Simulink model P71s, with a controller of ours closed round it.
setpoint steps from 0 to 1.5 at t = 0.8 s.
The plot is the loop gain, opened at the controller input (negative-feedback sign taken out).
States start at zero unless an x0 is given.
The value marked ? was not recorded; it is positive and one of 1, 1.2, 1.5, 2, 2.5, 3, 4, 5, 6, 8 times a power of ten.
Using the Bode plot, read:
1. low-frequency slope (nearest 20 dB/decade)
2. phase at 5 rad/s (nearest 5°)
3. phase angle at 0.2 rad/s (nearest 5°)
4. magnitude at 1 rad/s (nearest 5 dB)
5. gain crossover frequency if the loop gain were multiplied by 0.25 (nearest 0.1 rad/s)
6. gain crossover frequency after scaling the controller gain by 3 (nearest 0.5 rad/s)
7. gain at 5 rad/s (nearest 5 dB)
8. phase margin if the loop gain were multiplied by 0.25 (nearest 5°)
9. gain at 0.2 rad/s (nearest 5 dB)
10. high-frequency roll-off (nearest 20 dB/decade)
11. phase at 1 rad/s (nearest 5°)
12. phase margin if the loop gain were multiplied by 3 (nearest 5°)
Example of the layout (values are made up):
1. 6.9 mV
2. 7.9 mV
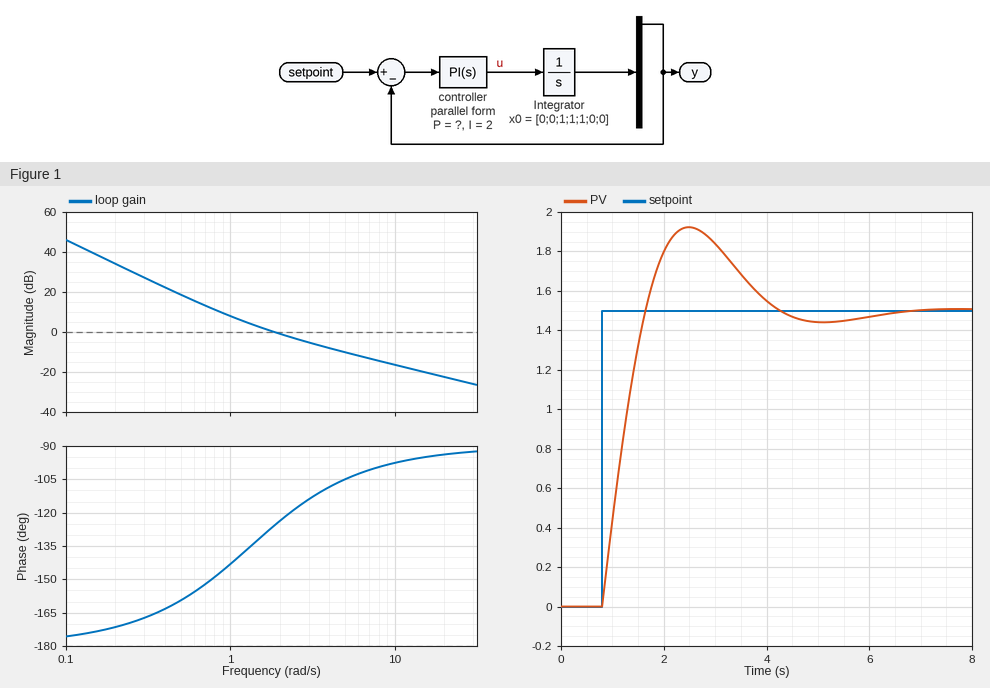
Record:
1. -40 dB/decade
2. -105°
3. -170°
4. 10 dB
5. 0.8 rad/s
6. 4.5 rad/s
7. -10 dB
8. 30°
9. 35 dB
10. -20 dB/decade
11. -145°
12. 75°
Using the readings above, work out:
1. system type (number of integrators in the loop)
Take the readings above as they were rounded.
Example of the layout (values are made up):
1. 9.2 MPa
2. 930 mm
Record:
1. 2
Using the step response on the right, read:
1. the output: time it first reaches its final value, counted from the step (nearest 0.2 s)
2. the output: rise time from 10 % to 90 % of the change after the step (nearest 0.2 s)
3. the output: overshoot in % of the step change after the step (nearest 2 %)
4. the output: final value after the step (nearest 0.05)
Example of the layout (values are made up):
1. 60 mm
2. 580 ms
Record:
1. 0.8 s
2. 0.6 s
3. 28 %
4. 1.50
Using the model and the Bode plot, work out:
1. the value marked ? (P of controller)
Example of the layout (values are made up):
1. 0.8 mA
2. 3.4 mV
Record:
1. 1.5
